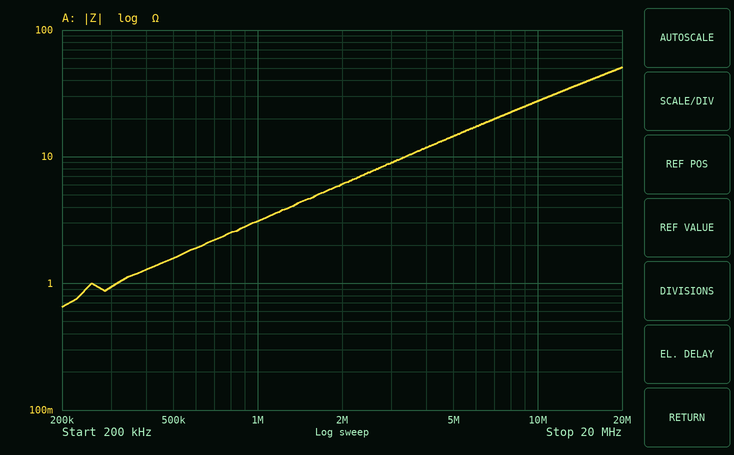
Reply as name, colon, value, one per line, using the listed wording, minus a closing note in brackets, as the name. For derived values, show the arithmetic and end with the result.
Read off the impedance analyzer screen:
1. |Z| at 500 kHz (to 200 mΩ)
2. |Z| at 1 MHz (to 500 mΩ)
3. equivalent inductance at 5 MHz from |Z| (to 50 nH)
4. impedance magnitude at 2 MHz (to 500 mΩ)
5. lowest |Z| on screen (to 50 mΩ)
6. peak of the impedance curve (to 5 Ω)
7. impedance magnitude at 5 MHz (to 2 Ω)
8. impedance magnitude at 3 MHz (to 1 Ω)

|Z| at 500 kHz: 1.6 Ω
|Z| at 1 MHz: 3.0 Ω
equivalent inductance at 5 MHz from |Z|: L = 14 Ω/(2π × 5 MHz) ≈ 446 nH, so 450 nH to the nearest 50 nH
impedance magnitude at 2 MHz: 6.0 Ω
lowest |Z| on screen: 650 mΩ
peak of the impedance curve: 50 Ω
impedance magnitude at 5 MHz: 14 Ω
impedance magnitude at 3 MHz: 9 Ω
